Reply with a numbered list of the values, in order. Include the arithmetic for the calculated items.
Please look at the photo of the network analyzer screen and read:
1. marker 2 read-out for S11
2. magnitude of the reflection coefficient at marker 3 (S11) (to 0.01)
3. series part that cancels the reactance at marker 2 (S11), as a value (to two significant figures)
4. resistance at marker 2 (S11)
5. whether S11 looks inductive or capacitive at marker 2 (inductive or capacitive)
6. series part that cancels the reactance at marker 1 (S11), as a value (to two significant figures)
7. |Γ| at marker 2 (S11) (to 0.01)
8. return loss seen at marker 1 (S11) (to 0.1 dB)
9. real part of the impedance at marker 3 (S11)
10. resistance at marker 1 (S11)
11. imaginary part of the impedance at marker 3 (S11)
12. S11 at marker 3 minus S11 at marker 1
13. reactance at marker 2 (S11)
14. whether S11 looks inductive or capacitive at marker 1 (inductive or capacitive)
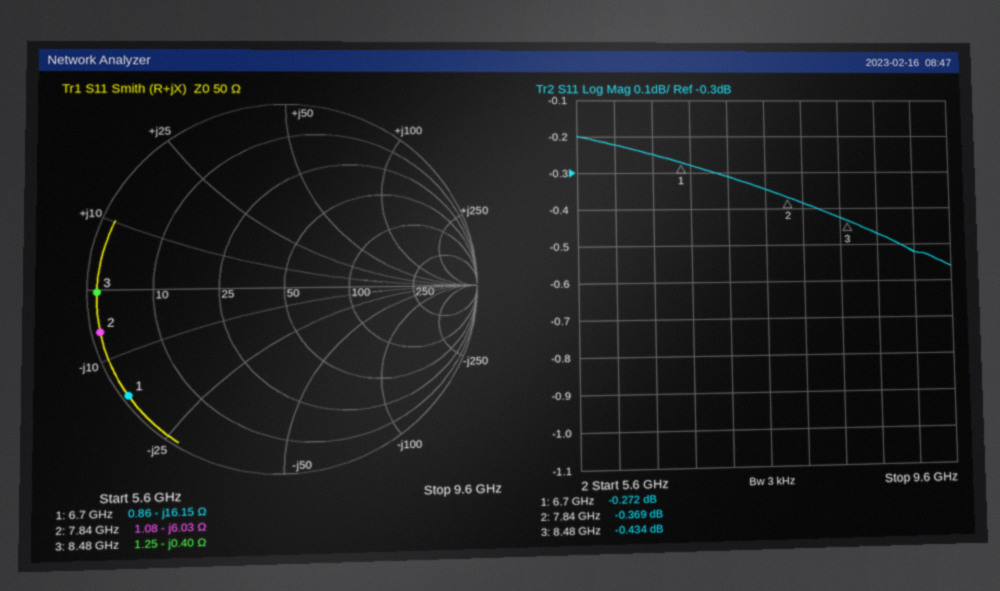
1. -0.369 dB
2. 0.95
3. L = 6.03 Ω/(2π × 7.84 GHz) ≈ 122 pH, so 120 pH to two significant figures
4. 1.08 Ω
5. capacitive
6. L = 16.15 Ω/(2π × 6.7 GHz) ≈ 384 pH, so 380 pH to two significant figures
7. 0.96
8. 0.3 dB
9. 1.25 Ω
10. 0.86 Ω
11. -0.40 Ω
12. -0.434 − (-0.272) = -0.162 dB
13. -6.03 Ω
14. capacitive
